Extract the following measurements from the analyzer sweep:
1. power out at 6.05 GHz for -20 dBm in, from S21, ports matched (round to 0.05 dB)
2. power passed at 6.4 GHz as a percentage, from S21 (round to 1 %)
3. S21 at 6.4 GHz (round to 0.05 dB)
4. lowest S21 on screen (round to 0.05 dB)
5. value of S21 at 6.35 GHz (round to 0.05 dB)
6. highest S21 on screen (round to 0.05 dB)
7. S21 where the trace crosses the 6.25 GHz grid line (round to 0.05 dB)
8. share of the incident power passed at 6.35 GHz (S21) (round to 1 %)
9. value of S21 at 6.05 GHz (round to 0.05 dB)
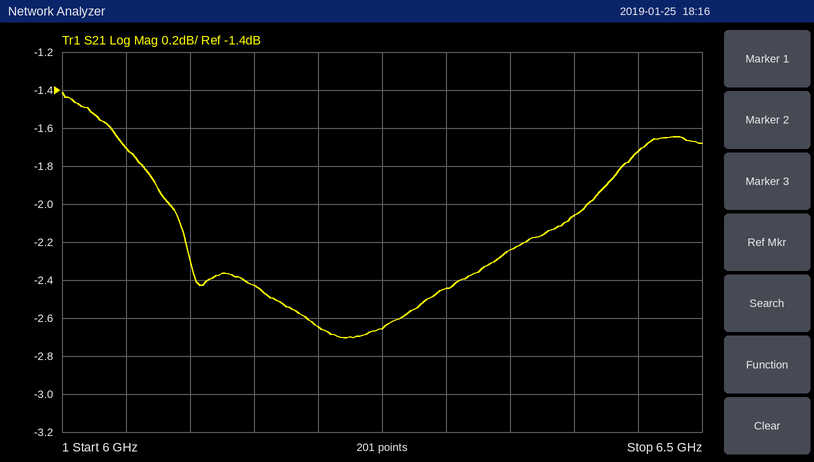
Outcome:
-21.70 dBm
62 %
-2.05 dB
-2.70 dB
-2.25 dB
-1.40 dB
-2.65 dB
60 %
-1.70 dB
